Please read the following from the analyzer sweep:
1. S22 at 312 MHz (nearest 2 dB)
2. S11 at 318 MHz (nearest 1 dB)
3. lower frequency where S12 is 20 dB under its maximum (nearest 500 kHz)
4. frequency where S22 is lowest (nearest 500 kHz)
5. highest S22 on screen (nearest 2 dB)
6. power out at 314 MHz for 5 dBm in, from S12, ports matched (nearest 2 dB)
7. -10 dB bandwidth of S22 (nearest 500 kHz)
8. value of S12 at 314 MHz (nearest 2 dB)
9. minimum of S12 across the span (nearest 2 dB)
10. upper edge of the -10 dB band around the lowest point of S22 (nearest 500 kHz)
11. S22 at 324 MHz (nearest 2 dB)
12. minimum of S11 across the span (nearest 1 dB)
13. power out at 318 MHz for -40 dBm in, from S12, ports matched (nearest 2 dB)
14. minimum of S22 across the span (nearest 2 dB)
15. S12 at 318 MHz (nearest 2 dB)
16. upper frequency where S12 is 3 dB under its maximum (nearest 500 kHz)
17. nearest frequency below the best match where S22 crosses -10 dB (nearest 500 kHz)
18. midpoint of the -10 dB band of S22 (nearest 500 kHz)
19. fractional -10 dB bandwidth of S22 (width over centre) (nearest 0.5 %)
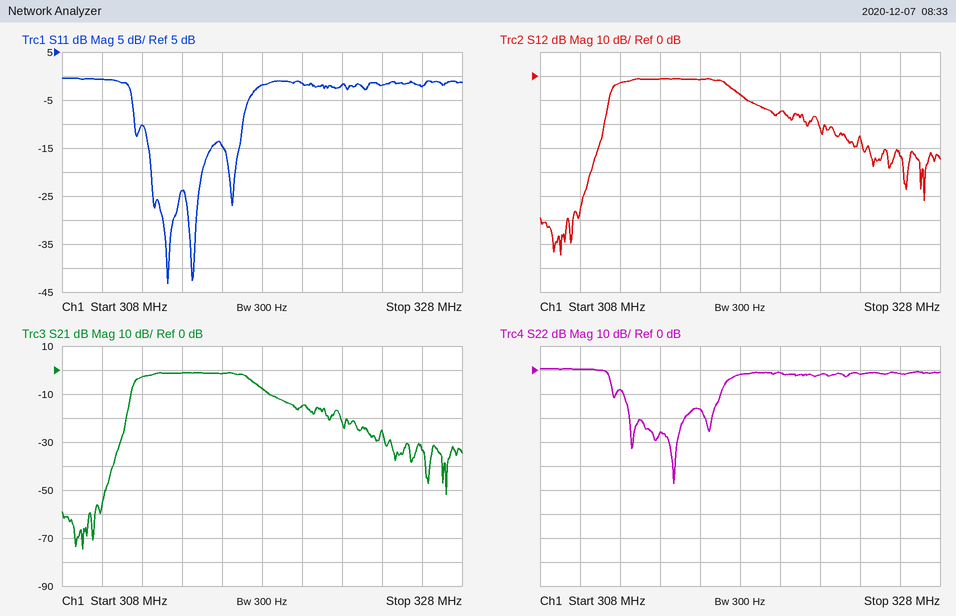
-8 dB
-2 dB
311.0 MHz
314.5 MHz
0 dB
4 dBm
5.0 MHz
-2 dB
-74 dB
317.0 MHz
-2 dB
-43 dB
-48 dBm
-48 dB
-8 dB
317.5 MHz
312.0 MHz
314.5 MHz
1.5 %
